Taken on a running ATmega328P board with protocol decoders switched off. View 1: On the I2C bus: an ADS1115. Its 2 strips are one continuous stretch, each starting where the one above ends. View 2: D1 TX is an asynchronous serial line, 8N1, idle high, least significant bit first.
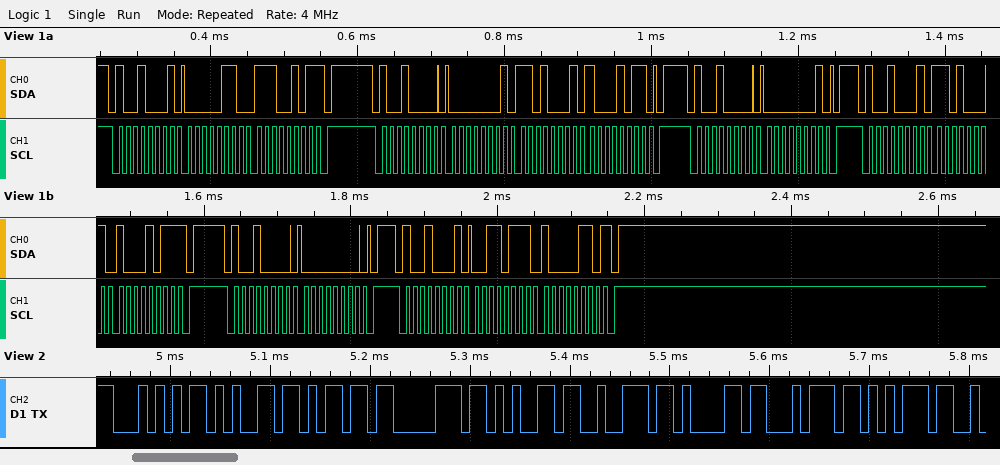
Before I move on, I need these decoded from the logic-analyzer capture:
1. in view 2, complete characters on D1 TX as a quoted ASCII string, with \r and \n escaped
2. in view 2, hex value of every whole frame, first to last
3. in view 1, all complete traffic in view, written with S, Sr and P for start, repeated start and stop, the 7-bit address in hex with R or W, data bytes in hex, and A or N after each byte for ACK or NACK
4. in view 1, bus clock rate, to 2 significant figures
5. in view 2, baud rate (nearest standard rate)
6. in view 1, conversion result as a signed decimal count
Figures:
"Temperatu"
54 65 6D 70 65 72 61 74 75
S 48R A 06 A E5 N P S 48W A 01 A D1 A 8B A P S 48W A 01 A P S 48R A D1 A 8B N P S 48W A 00 A P S 48R A 37 A 86 N P
100 kHz
115200 baud
14214
